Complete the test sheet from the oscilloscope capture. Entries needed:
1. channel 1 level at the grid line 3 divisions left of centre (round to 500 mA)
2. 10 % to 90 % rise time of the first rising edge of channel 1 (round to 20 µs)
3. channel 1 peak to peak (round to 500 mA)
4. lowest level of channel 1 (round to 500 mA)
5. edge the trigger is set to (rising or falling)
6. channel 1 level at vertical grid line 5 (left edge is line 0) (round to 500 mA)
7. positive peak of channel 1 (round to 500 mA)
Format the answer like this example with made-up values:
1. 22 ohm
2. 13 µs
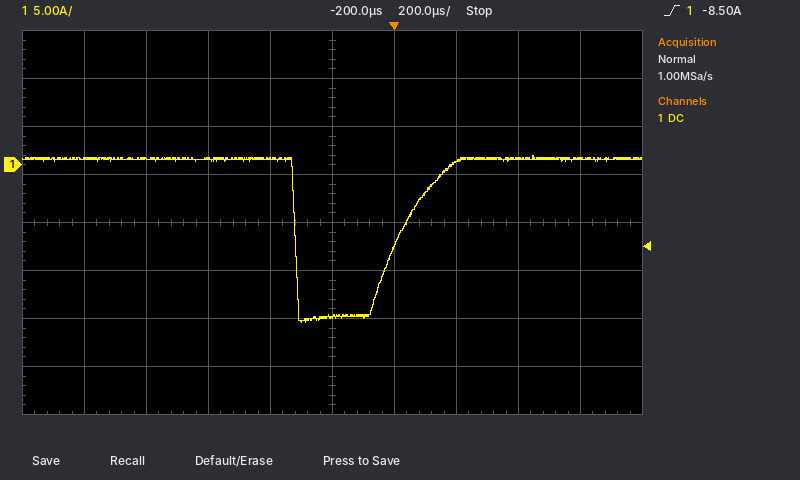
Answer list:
1. 500 mA
2. 220 µs
3. 17.5 A
4. -16.5 A
5. rising
6. -16.0 A
7. 1.0 A
